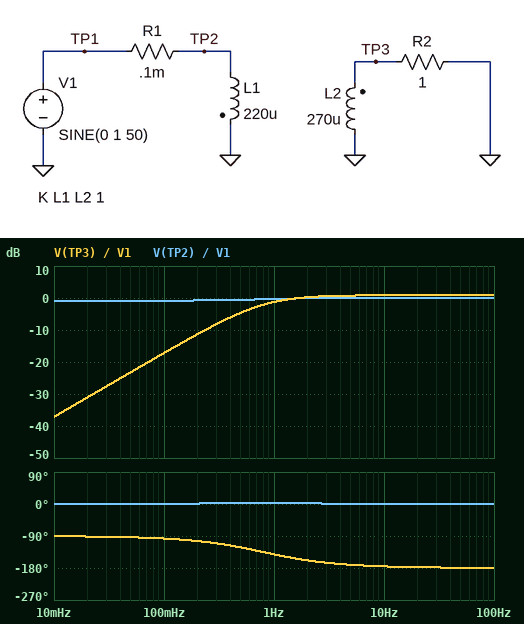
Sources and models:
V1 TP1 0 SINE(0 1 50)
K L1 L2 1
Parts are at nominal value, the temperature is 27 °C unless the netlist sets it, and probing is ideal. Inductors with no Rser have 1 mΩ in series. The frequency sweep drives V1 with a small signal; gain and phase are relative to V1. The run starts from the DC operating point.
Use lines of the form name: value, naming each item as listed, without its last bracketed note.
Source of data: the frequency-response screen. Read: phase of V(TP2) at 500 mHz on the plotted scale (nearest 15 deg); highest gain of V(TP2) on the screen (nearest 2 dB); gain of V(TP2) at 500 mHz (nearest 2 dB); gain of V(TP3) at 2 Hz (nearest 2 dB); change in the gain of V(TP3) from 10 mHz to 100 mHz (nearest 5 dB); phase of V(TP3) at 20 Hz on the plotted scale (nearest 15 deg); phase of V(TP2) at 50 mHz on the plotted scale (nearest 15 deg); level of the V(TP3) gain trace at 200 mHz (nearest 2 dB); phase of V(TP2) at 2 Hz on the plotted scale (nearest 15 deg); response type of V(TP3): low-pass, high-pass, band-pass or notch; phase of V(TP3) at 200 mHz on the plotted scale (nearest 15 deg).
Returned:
phase of V(TP2) at 500 mHz on the plotted scale: 0 deg
highest gain of V(TP2) on the screen: 0 dB
gain of V(TP2) at 500 mHz: 0 dB
gain of V(TP3) at 2 Hz: 0 dB
change in the gain of V(TP3) from 10 mHz to 100 mHz: 20 dB
phase of V(TP3) at 20 Hz on the plotted scale: -180 deg
phase of V(TP2) at 50 mHz on the plotted scale: 0 deg
level of the V(TP3) gain trace at 200 mHz: -12 dB
phase of V(TP2) at 2 Hz on the plotted scale: 0 deg
response type of V(TP3): low-pass, high-pass, band-pass or notch: high-pass
phase of V(TP3) at 200 mHz on the plotted scale: -105 deg
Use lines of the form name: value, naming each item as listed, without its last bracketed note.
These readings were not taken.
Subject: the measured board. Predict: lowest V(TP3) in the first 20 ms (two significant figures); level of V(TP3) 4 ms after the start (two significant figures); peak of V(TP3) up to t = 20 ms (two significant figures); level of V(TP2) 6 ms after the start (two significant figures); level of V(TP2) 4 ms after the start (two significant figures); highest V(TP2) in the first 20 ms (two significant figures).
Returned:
lowest V(TP3) in the first 20 ms: -1.1 V
level of V(TP3) 4 ms after the start: -1.0 V
peak of V(TP3) up to t = 20 ms: 1.1 V
level of V(TP2) 6 ms after the start: 950 mV
level of V(TP2) 4 ms after the start: 950 mV
highest V(TP2) in the first 20 ms: 1.0 V
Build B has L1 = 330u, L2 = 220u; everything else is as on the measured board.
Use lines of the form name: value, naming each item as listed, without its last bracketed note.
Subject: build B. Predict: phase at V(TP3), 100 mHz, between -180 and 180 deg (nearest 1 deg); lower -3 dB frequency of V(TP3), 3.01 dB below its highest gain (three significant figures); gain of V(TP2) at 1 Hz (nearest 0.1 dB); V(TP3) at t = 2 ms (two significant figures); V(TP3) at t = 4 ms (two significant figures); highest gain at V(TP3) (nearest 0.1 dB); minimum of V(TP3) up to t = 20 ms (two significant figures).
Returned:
phase at V(TP3), 100 mHz, between -180 and 180 deg: -101 deg
lower -3 dB frequency of V(TP3), 3.01 dB below its highest gain: 530 mHz
gain of V(TP2) at 1 Hz: -0.2 dB
V(TP3) at t = 2 ms: -480 mV
V(TP3) at t = 4 ms: -770 mV
highest gain at V(TP3): -1.8 dB
minimum of V(TP3) up to t = 20 ms: -810 mV
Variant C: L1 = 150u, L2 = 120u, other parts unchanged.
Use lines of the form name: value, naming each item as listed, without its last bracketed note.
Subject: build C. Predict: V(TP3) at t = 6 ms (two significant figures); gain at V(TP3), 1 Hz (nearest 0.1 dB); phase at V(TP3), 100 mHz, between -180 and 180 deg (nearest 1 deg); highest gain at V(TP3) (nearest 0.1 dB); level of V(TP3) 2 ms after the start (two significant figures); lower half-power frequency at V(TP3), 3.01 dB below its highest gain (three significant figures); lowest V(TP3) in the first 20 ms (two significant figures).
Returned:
V(TP3) at t = 6 ms: -820 mV
gain at V(TP3), 1 Hz: -4.7 dB
phase at V(TP3), 100 mHz, between -180 and 180 deg: -95 deg
highest gain at V(TP3): -1.0 dB
level of V(TP3) 2 ms after the start: -520 mV
lower half-power frequency at V(TP3), 3.01 dB below its highest gain: 1.17 Hz
lowest V(TP3) in the first 20 ms: -870 mV
